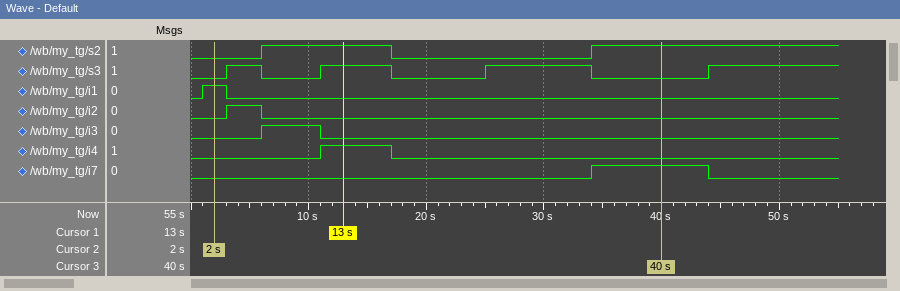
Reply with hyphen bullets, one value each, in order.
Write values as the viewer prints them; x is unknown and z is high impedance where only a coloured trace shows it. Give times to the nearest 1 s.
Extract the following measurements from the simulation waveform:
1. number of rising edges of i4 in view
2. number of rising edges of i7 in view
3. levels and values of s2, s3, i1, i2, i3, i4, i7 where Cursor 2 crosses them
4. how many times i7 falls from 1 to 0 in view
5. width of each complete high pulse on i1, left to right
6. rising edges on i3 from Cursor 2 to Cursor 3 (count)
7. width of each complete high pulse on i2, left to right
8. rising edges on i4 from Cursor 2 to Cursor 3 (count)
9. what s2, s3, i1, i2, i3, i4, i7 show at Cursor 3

- 1
- 1
- s2=0, s3=0, i1=1, i2=0, i3=0, i4=0, i7=0
- 1
- 2 s
- 1
- 3 s
- 1
- s2=1, s3=0, i1=0, i2=0, i3=0, i4=0, i7=1
